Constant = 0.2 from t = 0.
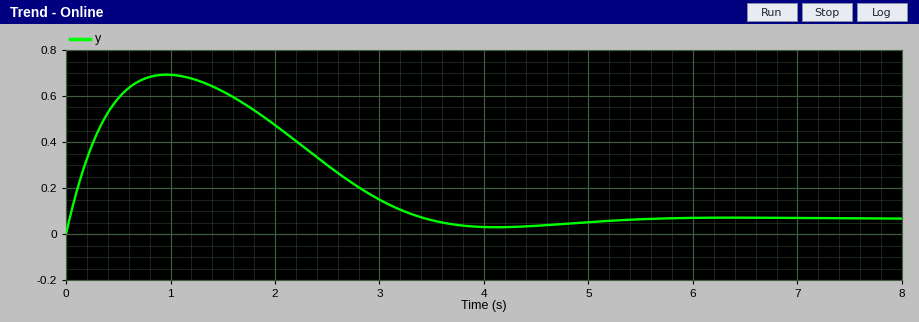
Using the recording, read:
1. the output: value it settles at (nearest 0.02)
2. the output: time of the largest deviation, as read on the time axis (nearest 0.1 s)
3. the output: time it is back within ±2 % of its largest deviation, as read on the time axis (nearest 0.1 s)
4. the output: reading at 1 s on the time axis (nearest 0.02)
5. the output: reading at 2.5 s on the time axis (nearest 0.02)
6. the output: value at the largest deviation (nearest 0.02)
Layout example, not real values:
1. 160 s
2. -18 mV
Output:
1. 0.06
2. 1.0 s
3. 5.1 s
4. 0.70
5. 0.30
6. 0.70
